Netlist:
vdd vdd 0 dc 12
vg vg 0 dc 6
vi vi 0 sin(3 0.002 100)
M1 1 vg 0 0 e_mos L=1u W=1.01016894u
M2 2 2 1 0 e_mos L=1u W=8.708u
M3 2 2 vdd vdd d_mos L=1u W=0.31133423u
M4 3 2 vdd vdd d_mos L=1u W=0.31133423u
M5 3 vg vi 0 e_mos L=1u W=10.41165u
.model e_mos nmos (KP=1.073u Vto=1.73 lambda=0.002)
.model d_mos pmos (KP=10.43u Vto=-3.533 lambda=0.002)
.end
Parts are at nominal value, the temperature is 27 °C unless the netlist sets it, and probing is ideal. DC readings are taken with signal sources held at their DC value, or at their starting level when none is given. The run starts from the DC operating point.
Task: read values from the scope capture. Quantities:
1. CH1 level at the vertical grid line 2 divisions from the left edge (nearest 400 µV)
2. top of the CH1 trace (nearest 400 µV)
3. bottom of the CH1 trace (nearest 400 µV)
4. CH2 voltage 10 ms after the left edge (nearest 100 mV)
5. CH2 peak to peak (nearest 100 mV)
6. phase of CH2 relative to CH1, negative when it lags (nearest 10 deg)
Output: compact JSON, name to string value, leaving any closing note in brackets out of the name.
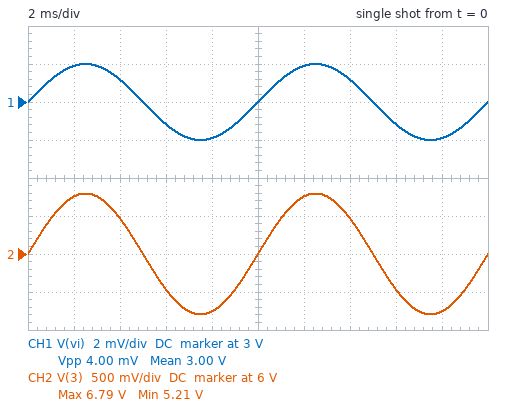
{"CH1 level at the vertical grid line 2 divisions from the left edge": "3.0012 V", "top of the CH1 trace": "3.0020 V", "bottom of the CH1 trace": "2.9980 V", "CH2 voltage 10 ms after the left edge": "6.0 V", "CH2 peak to peak": "1.6 V", "phase of CH2 relative to CH1, negative when it lags": "0 deg"}
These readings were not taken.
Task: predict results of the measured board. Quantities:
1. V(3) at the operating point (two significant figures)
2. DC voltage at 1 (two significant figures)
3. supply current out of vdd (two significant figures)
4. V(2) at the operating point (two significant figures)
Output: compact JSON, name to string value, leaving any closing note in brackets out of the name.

{"V(3) at the operating point": "6.0 V", "DC voltage at 1": "3.0 V", "supply current out of vdd": "18 µA", "V(2) at the operating point": "6.1 V"}
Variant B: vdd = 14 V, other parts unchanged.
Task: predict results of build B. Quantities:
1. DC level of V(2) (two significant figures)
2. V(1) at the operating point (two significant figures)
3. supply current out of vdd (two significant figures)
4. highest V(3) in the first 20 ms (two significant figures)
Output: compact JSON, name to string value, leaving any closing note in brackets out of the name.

{"DC level of V(2)": "8.0 V", "V(1) at the operating point": "4.8 V", "supply current out of vdd": "19 µA", "highest V(3) in the first 20 ms": "12 V"}
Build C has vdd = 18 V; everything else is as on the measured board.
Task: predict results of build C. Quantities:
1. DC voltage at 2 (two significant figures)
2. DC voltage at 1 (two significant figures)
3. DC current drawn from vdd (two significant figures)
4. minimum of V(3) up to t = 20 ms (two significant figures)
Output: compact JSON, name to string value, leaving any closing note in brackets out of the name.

{"DC voltage at 2": "12 V", "DC voltage at 1": "8.8 V", "DC current drawn from vdd": "19 µA", "minimum of V(3) up to t = 20 ms": "16 V"}
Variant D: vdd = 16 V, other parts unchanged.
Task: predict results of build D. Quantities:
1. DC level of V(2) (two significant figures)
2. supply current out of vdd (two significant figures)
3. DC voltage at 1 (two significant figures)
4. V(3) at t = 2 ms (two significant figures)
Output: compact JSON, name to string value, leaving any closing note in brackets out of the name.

{"DC level of V(2)": "10 V", "supply current out of vdd": "19 µA", "DC voltage at 1": "6.8 V", "V(3) at t = 2 ms": "14 V"}
